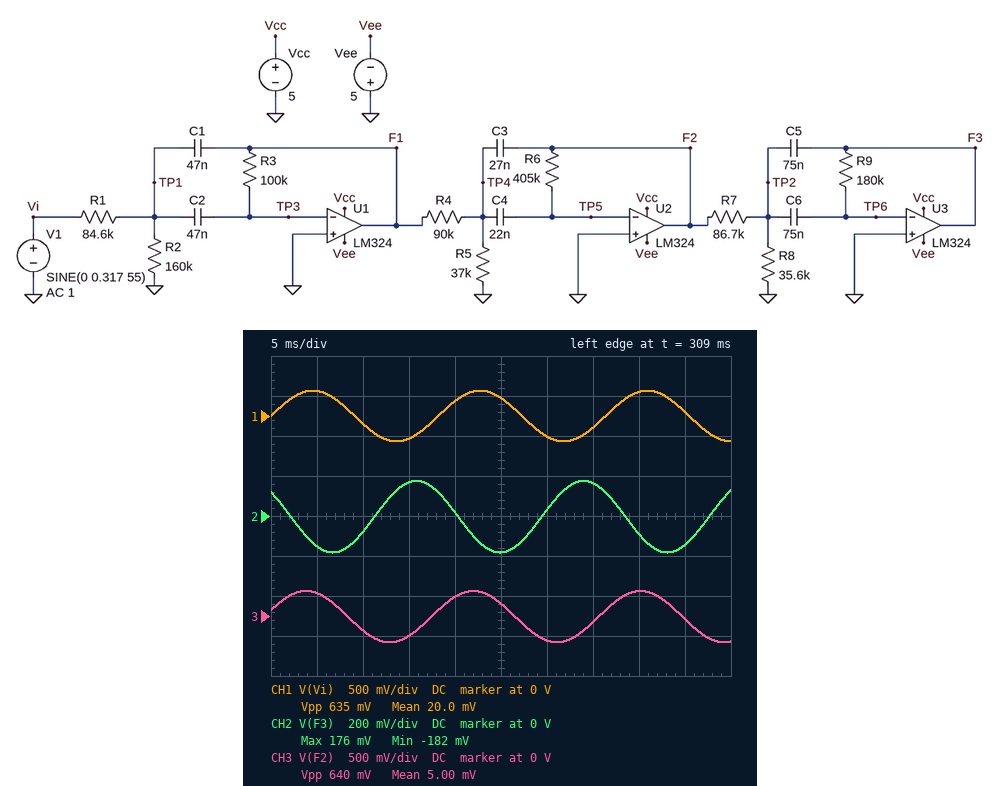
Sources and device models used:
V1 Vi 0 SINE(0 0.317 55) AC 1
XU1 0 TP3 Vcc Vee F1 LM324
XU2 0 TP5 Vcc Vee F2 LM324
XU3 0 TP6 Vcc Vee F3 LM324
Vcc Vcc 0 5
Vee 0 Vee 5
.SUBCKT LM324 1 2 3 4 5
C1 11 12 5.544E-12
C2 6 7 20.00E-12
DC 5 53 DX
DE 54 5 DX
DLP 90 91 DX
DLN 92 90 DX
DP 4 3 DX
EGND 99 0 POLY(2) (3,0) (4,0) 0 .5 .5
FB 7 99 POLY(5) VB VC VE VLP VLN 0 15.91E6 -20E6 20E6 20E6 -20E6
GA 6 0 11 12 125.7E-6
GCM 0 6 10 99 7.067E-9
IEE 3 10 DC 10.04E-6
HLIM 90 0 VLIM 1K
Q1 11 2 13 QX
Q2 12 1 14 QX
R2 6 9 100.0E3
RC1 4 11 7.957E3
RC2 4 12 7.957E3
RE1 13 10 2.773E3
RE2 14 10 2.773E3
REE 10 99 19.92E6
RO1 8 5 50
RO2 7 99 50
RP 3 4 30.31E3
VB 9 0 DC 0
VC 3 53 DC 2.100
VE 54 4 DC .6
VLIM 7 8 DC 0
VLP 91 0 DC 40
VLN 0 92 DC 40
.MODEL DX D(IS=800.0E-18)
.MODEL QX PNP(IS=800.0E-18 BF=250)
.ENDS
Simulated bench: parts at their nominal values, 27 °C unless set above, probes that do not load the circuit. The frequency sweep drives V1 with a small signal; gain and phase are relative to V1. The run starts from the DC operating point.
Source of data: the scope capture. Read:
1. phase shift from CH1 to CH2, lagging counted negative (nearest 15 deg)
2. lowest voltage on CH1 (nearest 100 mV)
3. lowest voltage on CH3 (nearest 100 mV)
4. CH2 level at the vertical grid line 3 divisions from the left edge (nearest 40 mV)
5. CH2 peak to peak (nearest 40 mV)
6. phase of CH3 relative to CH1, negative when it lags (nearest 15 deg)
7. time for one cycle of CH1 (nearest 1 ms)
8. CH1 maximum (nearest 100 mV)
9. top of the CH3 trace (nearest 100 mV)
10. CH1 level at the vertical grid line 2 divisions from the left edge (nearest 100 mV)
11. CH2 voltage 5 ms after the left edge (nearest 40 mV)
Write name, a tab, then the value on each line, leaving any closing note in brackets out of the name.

phase shift from CH1 to CH2, lagging counted negative	135 deg
lowest voltage on CH1	-300 mV
lowest voltage on CH3	-300 mV
CH2 level at the vertical grid line 3 divisions from the left edge	160 mV
CH2 peak to peak	360 mV
phase of CH3 relative to CH1, negative when it lags	15 deg
time for one cycle of CH1	18 ms
CH1 maximum	300 mV
top of the CH3 trace	300 mV
CH1 level at the vertical grid line 2 divisions from the left edge	-100 mV
CH2 voltage 5 ms after the left edge	-160 mV
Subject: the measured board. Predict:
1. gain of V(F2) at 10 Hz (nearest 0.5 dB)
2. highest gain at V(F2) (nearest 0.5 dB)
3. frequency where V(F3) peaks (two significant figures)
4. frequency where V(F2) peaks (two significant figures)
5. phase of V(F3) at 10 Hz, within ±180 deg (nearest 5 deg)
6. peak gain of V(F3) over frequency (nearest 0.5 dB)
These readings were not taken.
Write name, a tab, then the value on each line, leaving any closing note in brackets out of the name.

gain of V(F2) at 10 Hz	-30.0 dB
highest gain at V(F2)	1.0 dB
frequency where V(F3) peaks	55 Hz
frequency where V(F2) peaks	61 Hz
phase of V(F3) at 10 Hz, within ±180 deg	50 deg
peak gain of V(F3) over frequency	-5.0 dB
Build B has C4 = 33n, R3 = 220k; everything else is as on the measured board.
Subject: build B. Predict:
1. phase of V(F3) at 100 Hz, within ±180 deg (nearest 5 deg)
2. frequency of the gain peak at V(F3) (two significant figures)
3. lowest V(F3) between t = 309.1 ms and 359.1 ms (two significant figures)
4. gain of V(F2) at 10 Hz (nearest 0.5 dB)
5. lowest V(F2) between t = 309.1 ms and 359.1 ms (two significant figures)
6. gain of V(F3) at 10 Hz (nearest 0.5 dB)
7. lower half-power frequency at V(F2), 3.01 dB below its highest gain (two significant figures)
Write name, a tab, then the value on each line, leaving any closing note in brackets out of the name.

phase of V(F3) at 100 Hz, within ±180 deg	-35 deg
frequency of the gain peak at V(F3)	39 Hz
lowest V(F3) between t = 309.1 ms and 359.1 ms	-350 mV
gain of V(F2) at 10 Hz	-19.0 dB
lowest V(F2) between t = 309.1 ms and 359.1 ms	-630 mV
gain of V(F3) at 10 Hz	-30.5 dB
lower half-power frequency at V(F2), 3.01 dB below its highest gain	34 Hz
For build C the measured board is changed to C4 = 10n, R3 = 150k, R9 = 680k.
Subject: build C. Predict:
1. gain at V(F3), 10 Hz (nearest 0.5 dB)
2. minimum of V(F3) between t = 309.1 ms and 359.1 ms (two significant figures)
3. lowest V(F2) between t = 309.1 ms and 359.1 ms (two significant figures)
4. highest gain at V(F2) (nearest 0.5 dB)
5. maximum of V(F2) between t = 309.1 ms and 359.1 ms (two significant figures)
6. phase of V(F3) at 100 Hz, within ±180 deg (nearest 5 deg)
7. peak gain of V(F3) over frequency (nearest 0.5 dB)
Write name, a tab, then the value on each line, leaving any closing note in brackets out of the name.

gain at V(F3), 10 Hz	-30.0 dB
minimum of V(F3) between t = 309.1 ms and 359.1 ms	-76 mV
lowest V(F2) between t = 309.1 ms and 359.1 ms	-140 mV
highest gain at V(F2)	-5.0 dB
maximum of V(F2) between t = 309.1 ms and 359.1 ms	120 mV
phase of V(F3) at 100 Hz, within ±180 deg	20 deg
peak gain of V(F3) over frequency	-12.0 dB
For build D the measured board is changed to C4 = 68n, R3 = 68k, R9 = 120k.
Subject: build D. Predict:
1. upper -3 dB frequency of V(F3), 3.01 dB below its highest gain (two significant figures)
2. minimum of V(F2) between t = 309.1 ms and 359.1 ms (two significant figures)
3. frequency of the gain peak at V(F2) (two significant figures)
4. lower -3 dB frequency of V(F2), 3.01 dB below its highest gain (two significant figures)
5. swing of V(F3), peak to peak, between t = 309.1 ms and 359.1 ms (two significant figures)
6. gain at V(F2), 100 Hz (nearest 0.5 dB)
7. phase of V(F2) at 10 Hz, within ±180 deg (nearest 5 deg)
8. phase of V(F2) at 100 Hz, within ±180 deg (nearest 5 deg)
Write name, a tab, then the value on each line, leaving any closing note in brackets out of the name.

upper -3 dB frequency of V(F3), 3.01 dB below its highest gain	47 Hz
minimum of V(F2) between t = 309.1 ms and 359.1 ms	-230 mV
frequency of the gain peak at V(F2)	37 Hz
lower -3 dB frequency of V(F2), 3.01 dB below its highest gain	29 Hz
swing of V(F3), peak to peak, between t = 309.1 ms and 359.1 ms	240 mV
gain at V(F2), 100 Hz	-12.5 dB
phase of V(F2) at 10 Hz, within ±180 deg	150 deg
phase of V(F2) at 100 Hz, within ±180 deg	-110 deg
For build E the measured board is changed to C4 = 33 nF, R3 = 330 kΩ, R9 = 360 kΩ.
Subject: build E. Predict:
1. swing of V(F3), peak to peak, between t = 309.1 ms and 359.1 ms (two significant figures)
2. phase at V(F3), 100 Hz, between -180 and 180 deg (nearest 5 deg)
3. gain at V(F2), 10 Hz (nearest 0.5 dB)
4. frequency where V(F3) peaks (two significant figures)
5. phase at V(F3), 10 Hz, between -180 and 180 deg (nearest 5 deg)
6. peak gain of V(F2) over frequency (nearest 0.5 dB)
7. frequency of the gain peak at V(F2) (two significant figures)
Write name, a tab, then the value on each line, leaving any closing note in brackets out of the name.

swing of V(F3), peak to peak, between t = 309.1 ms and 359.1 ms	650 mV
phase at V(F3), 100 Hz, between -180 and 180 deg	-50 deg
gain at V(F2), 10 Hz	-15.0 dB
frequency where V(F3) peaks	25 Hz
phase at V(F3), 10 Hz, between -180 and 180 deg	45 deg
peak gain of V(F2) over frequency	7.5 dB
frequency of the gain peak at V(F2)	47 Hz
